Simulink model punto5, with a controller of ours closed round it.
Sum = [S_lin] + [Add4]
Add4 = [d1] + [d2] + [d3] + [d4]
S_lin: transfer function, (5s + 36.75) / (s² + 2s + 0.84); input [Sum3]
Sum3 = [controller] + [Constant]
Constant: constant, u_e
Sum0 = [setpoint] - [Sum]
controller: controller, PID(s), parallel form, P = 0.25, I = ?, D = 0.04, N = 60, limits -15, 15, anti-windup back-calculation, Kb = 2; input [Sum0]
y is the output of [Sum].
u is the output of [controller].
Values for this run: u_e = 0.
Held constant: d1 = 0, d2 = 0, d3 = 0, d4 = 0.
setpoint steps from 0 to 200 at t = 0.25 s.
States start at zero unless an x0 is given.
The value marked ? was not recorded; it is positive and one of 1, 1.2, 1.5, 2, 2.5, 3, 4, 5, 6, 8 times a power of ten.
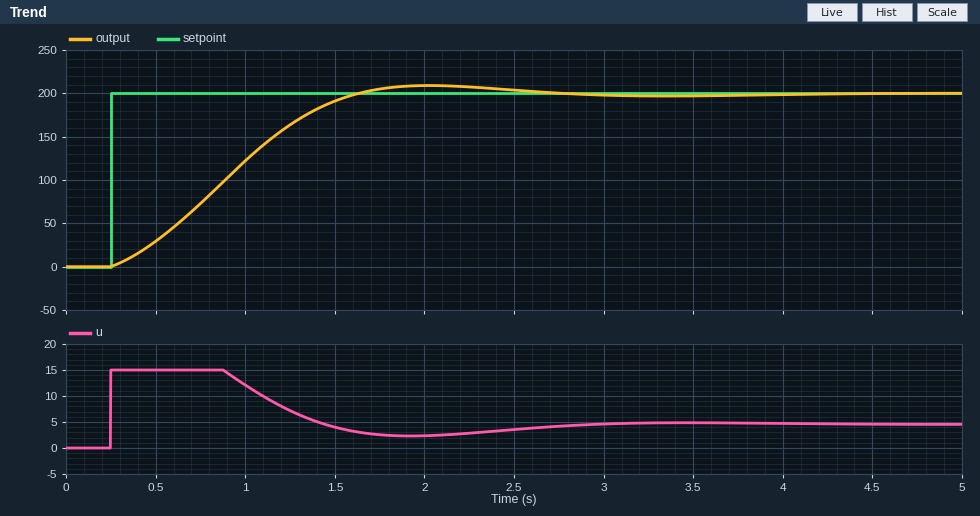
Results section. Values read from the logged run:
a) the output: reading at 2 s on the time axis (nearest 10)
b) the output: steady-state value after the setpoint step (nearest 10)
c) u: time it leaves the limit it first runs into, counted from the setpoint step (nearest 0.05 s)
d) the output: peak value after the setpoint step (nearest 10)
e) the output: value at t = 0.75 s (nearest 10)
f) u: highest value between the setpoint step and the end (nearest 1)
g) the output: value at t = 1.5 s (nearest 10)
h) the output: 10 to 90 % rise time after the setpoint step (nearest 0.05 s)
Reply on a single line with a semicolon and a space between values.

210; 200; 0.65 s; 210; 70; 15; 190; 0.95 s
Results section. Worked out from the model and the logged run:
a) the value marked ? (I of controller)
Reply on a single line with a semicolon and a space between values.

0.25
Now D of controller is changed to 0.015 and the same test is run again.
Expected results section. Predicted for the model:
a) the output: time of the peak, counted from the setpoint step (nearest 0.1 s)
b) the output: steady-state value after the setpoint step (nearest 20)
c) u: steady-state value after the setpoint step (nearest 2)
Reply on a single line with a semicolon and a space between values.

1.6 s; 200; 4
